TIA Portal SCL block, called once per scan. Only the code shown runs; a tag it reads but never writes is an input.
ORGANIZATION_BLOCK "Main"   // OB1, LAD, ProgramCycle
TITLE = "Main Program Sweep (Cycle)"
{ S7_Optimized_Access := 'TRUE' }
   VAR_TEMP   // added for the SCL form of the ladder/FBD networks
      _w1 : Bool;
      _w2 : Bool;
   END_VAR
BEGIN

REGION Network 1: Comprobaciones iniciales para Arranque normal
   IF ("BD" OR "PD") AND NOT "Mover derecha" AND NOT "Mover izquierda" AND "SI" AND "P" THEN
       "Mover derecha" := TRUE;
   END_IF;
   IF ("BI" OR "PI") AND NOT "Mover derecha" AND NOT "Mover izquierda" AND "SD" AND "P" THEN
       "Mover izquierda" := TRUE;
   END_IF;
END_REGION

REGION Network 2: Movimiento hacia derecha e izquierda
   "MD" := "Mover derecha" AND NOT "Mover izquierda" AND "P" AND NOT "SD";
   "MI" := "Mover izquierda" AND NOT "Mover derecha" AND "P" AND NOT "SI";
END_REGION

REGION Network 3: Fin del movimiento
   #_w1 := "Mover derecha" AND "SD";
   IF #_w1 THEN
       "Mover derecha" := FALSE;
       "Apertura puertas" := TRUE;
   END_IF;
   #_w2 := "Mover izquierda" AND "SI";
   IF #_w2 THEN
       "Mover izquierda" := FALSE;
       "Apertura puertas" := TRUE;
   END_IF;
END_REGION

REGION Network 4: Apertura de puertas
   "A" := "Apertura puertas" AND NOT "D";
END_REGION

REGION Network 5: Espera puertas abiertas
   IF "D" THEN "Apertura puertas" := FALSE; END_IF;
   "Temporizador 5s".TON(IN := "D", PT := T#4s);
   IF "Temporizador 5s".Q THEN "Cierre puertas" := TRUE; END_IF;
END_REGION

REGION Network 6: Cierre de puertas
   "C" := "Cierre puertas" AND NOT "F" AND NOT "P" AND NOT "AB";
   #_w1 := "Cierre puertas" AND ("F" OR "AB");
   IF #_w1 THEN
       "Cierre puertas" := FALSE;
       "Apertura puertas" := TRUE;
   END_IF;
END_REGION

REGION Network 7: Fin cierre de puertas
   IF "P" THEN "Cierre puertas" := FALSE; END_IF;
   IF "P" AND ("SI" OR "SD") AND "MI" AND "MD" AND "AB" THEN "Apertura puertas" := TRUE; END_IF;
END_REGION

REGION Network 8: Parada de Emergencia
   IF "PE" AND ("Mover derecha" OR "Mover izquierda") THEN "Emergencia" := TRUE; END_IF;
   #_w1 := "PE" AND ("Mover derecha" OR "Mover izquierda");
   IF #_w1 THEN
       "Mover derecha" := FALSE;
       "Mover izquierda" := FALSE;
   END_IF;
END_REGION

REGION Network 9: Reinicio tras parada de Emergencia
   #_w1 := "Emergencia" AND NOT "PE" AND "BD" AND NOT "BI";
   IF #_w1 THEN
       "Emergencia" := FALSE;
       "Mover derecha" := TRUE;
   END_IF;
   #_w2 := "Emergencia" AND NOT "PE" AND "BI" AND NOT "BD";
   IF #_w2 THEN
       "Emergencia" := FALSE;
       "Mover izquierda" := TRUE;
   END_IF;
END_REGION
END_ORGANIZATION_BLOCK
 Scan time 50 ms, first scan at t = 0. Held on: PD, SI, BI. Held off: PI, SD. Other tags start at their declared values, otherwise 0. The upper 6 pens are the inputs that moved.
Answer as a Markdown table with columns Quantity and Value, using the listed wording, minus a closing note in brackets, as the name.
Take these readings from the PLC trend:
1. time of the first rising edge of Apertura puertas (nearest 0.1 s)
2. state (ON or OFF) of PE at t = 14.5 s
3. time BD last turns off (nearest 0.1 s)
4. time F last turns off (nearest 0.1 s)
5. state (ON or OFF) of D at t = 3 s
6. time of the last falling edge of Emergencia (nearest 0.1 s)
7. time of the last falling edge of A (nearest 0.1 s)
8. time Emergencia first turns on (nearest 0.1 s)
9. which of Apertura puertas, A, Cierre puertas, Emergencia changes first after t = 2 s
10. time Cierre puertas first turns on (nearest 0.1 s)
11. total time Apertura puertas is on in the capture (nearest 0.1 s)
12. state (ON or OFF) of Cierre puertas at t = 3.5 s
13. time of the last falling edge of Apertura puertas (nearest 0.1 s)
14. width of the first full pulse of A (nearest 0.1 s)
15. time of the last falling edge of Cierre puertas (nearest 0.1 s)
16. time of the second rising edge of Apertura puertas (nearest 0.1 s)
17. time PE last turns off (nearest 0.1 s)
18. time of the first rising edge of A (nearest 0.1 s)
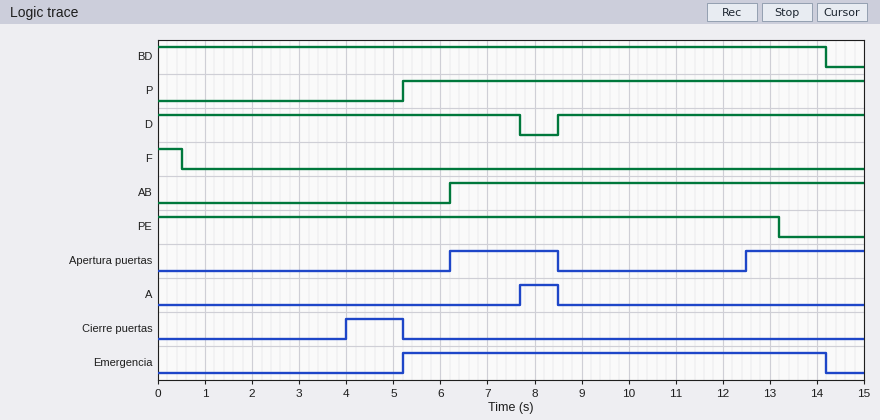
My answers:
| Quantity | Value |
|---|---|
| time of the first rising edge of Apertura puertas | 6.2 s |
| state (ON or OFF) of PE at t = 14.5 s | OFF |
| time BD last turns off | 14.2 s |
| time F last turns off | 0.5 s |
| state (ON or OFF) of D at t = 3 s | ON |
| time of the last falling edge of Emergencia | 14.2 s |
| time of the last falling edge of A | 8.5 s |
| time Emergencia first turns on | 5.2 s |
| which of Apertura puertas, A, Cierre puertas, Emergencia changes first after t = 2 s | Cierre puertas |
| time Cierre puertas first turns on | 4.0 s |
| total time Apertura puertas is on in the capture | 4.8 s |
| state (ON or OFF) of Cierre puertas at t = 3.5 s | OFF |
| time of the last falling edge of Apertura puertas | 8.5 s |
| width of the first full pulse of A | 0.8 s |
| time of the last falling edge of Cierre puertas | 5.2 s |
| time of the second rising edge of Apertura puertas | 12.5 s |
| time PE last turns off | 13.2 s |
| time of the first rising edge of A | 7.7 s |
